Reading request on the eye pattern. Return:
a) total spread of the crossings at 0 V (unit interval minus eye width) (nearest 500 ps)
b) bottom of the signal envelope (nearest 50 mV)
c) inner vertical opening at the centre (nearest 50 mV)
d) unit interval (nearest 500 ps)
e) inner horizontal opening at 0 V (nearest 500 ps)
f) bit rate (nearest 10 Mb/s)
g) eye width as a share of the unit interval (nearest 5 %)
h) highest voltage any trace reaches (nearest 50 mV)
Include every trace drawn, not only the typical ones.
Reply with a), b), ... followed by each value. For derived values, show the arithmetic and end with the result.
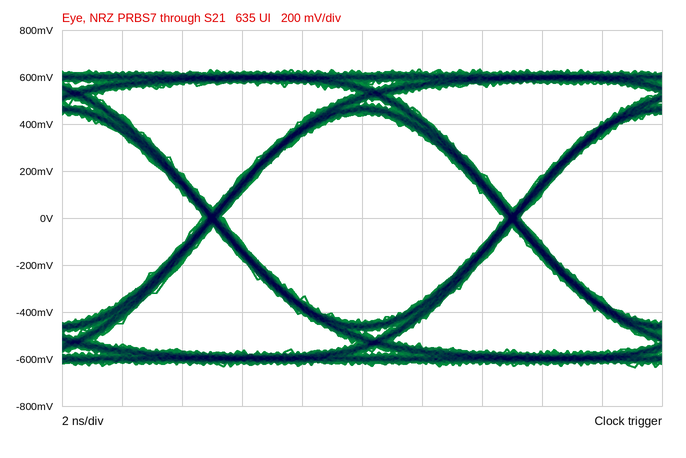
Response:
a) 500 ps
b) -650 mV
c) 900 mV
d) 10.0 ns
e) 9.5 ns
f) 100 Mb/s
g) 9.5 ns / 10.0 ns ≈ 95 %
h) 650 mV
